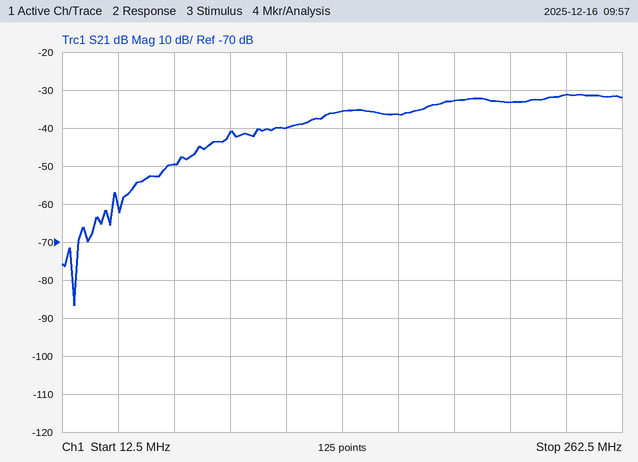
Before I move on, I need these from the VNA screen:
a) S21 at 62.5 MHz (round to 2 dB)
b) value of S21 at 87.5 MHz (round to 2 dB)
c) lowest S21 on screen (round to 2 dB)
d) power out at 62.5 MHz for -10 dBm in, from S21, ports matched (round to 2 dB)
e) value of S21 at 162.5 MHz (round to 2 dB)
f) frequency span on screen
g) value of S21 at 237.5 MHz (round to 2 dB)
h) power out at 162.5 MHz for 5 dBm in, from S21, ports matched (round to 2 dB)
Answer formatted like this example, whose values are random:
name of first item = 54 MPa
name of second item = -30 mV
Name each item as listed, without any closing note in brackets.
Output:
S21 at 62.5 MHz = -50 dB
value of S21 at 87.5 MHz = -42 dB
lowest S21 on screen = -86 dB
power out at 62.5 MHz for -10 dBm in, from S21, ports matched = -60 dBm
value of S21 at 162.5 MHz = -36 dB
frequency span on screen = 250 MHz
value of S21 at 237.5 MHz = -32 dB
power out at 162.5 MHz for 5 dBm in, from S21, ports matched = -32 dBm
